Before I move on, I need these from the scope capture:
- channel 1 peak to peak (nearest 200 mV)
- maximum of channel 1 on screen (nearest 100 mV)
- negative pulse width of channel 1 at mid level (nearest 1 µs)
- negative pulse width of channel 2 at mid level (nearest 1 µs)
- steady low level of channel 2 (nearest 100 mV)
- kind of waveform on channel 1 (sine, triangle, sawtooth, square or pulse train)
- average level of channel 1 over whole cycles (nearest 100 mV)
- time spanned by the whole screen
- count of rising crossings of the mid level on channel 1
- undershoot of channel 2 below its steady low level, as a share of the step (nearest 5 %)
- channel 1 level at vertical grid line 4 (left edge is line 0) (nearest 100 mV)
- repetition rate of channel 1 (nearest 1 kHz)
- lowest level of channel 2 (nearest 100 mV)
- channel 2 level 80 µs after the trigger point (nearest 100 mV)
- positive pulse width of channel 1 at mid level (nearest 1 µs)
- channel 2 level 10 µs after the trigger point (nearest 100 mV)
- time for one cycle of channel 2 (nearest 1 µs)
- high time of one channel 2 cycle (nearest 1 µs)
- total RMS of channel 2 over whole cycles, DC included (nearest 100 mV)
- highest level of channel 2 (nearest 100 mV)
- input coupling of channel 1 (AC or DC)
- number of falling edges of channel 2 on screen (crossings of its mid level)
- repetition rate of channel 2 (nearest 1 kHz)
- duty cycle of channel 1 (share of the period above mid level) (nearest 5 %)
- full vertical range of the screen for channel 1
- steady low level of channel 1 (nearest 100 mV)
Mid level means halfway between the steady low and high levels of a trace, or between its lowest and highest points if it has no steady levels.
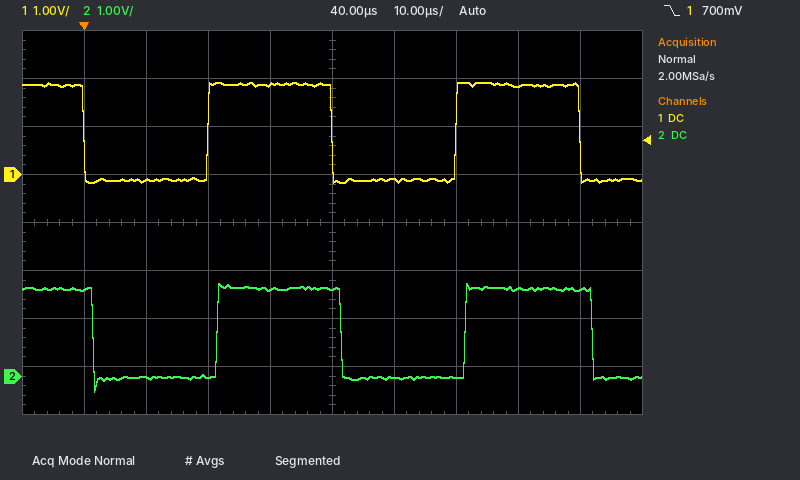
2.0 V
1.9 V
20 µs
20 µs
0.0 V
square
900 mV
100 µs
2
15 %
1.9 V
25 kHz
-300 mV
1.8 V
20 µs
0.0 V
40 µs
20 µs
1.3 V
1.9 V
DC
3
25 kHz
50 %
8 V
-100 mV
